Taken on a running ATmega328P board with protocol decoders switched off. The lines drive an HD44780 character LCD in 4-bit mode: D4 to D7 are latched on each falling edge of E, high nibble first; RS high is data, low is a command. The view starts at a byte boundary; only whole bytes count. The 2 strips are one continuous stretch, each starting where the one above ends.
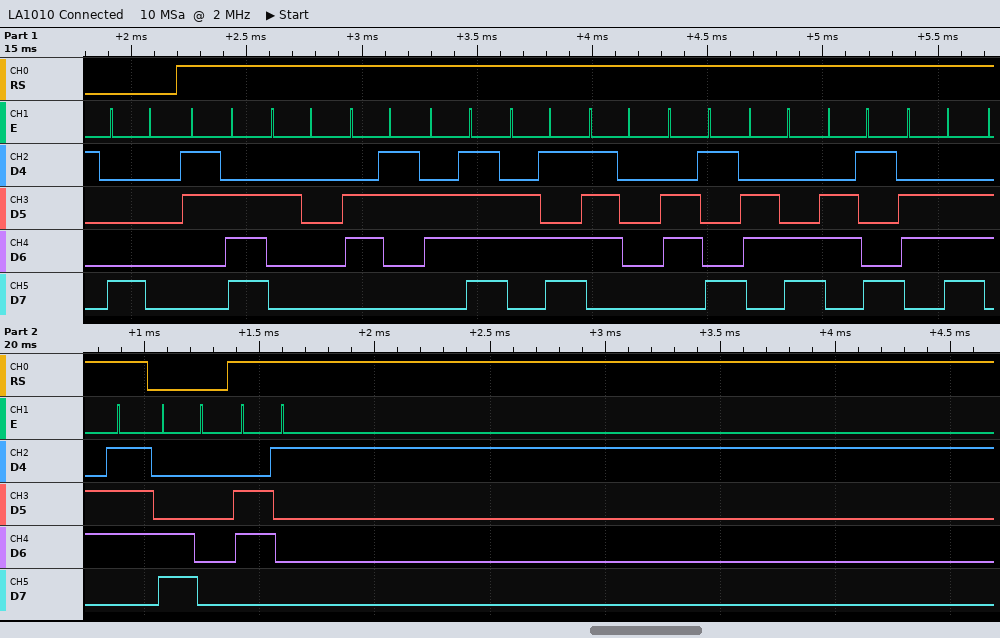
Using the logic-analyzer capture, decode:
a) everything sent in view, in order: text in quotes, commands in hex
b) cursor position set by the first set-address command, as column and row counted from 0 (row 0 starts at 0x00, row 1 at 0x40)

0x80 "> compiling" 0xC0 "a"
column 0, row 0
